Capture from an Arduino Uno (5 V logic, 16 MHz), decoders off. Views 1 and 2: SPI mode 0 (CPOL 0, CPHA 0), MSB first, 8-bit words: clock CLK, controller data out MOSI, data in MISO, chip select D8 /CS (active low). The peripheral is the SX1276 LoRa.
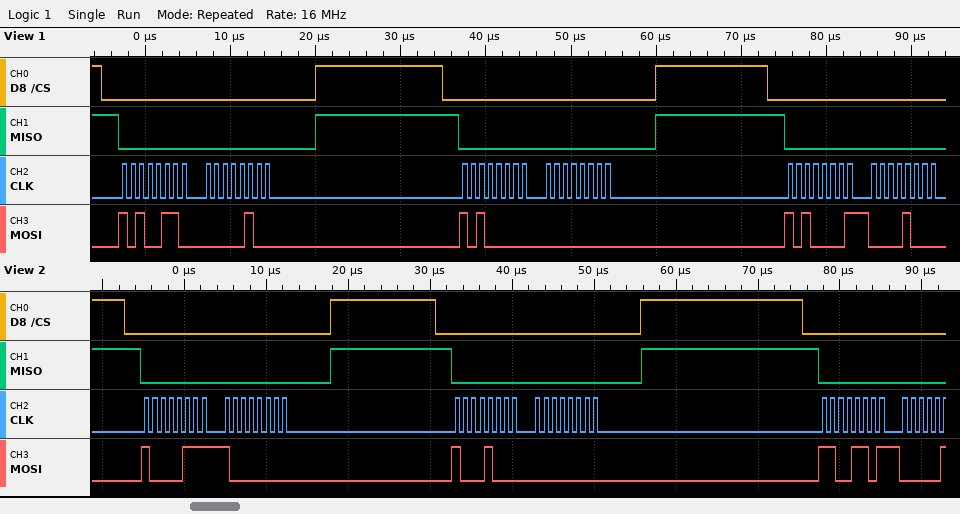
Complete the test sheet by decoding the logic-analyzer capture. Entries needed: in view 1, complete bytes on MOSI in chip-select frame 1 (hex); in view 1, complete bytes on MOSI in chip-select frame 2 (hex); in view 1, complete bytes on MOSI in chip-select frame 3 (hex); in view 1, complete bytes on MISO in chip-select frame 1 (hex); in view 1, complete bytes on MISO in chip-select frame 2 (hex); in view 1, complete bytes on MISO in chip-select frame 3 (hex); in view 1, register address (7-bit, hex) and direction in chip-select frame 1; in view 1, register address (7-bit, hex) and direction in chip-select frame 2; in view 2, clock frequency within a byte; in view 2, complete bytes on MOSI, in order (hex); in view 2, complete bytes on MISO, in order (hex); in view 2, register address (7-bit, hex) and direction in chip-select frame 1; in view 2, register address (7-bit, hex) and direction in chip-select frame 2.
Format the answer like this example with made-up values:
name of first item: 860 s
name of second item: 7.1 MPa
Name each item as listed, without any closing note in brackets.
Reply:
in view 1, complete bytes on MOSI in chip-select frame 1: A6 04
in view 1, complete bytes on MOSI in chip-select frame 2: A0 00
in view 1, complete bytes on MOSI in chip-select frame 3: A1 08
in view 1, complete bytes on MISO in chip-select frame 1: 00 00
in view 1, complete bytes on MISO in chip-select frame 2: 00 00
in view 1, complete bytes on MISO in chip-select frame 3: 00 00
in view 1, register address (7-bit, hex) and direction in chip-select frame 1: 0x26 write
in view 1, register address (7-bit, hex) and direction in chip-select frame 2: 0x20 write
in view 2, clock frequency within a byte: 1 MHz
in view 2, complete bytes on MOSI, in order: 87 80 88 00 CD
in view 2, complete bytes on MISO, in order: 00 00 00 00 00
in view 2, register address (7-bit, hex) and direction in chip-select frame 1: 0x07 write
in view 2, register address (7-bit, hex) and direction in chip-select frame 2: 0x08 write
